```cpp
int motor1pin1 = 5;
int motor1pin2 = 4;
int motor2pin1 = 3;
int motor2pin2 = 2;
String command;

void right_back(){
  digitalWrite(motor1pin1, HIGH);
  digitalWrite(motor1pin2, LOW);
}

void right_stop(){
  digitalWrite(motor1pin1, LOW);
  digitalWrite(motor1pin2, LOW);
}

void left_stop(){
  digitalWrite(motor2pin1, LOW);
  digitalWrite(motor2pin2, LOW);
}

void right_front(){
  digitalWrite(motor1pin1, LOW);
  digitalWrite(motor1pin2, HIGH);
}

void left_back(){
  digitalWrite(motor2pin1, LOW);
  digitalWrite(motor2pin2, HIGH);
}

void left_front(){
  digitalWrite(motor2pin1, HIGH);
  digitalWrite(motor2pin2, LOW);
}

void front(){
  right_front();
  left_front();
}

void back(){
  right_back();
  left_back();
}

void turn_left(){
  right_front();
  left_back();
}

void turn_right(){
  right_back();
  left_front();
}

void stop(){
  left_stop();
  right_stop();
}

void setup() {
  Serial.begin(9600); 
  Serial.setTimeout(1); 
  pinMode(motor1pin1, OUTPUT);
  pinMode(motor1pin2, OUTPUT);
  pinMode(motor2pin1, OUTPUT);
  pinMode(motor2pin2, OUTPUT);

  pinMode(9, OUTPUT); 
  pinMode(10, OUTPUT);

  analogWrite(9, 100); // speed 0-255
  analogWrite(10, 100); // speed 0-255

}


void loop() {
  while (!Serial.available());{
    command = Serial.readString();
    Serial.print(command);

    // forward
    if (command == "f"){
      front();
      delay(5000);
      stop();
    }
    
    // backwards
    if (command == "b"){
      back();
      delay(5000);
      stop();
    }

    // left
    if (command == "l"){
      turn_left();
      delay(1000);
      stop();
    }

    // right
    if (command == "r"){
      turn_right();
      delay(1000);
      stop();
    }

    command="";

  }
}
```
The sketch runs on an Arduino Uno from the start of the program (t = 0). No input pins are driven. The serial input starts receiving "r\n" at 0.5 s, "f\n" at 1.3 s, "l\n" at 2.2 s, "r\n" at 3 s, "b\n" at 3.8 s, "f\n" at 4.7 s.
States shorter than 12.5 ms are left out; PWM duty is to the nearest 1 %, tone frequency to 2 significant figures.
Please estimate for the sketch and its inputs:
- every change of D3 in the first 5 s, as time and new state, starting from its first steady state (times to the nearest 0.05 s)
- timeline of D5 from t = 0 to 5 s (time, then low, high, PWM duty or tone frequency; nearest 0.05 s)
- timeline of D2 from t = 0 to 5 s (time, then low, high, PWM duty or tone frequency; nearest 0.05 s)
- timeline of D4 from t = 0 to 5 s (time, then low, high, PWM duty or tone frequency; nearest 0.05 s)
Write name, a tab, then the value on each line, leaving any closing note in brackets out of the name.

every change of D3 in the first 5 s, as time and new state, starting from its first steady state	0 s low; 0.5 s high; 1.5 s low
timeline of D5 from t = 0 to 5 s	0 s low; 0.5 s high; 1.5 s low; 3.8 s high
timeline of D2 from t = 0 to 5 s	0 s low; 2.2 s high; 3.2 s low; 3.8 s high
timeline of D4 from t = 0 to 5 s	0 s low; 2.2 s high; 3.2 s low
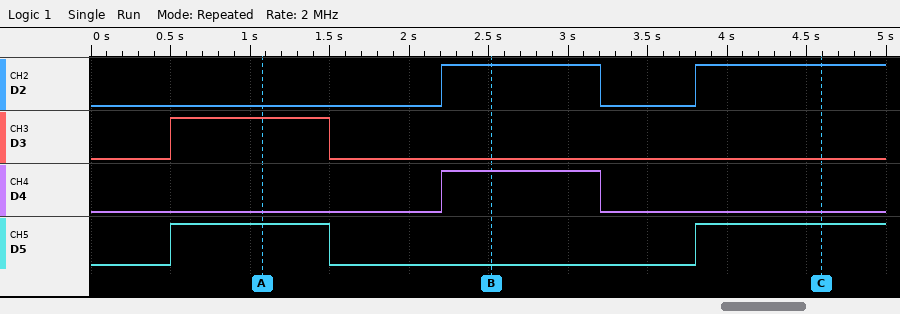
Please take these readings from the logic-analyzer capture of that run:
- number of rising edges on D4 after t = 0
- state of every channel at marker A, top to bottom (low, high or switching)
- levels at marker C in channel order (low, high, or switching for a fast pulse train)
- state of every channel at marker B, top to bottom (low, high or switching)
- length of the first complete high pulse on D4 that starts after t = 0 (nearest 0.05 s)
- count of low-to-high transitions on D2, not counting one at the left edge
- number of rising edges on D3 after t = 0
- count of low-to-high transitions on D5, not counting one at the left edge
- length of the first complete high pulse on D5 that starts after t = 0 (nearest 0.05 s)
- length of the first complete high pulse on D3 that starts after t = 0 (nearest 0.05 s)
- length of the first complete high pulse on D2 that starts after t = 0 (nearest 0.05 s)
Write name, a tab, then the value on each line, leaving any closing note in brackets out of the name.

number of rising edges on D4 after t = 0	1
state of every channel at marker A, top to bottom	D2 low, D3 high, D4 low, D5 high
levels at marker C in channel order	D2 high, D3 low, D4 low, D5 high
state of every channel at marker B, top to bottom	D2 high, D3 low, D4 high, D5 low
length of the first complete high pulse on D4 that starts after t = 0	1.00 s
count of low-to-high transitions on D2, not counting one at the left edge	2
number of rising edges on D3 after t = 0	1
count of low-to-high transitions on D5, not counting one at the left edge	2
length of the first complete high pulse on D5 that starts after t = 0	1.00 s
length of the first complete high pulse on D3 that starts after t = 0	1.00 s
length of the first complete high pulse on D2 that starts after t = 0	1.00 s
